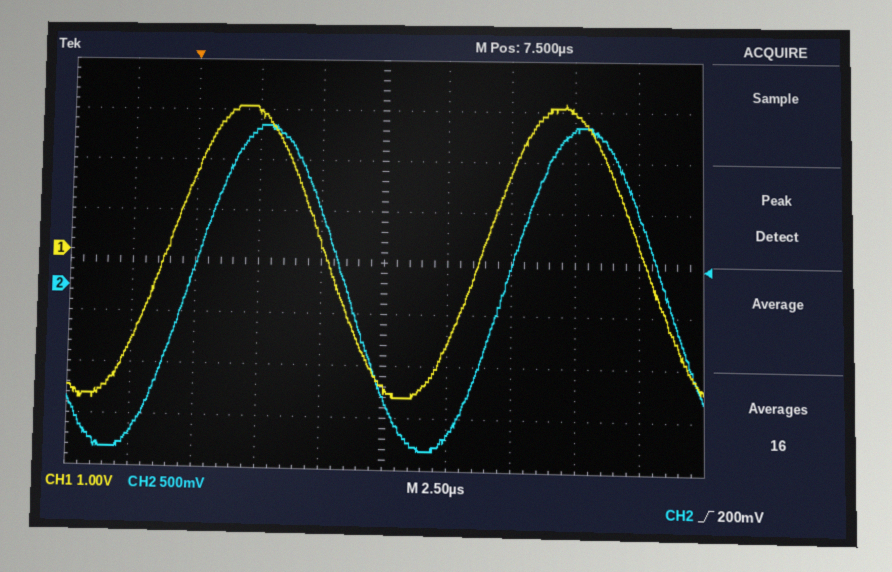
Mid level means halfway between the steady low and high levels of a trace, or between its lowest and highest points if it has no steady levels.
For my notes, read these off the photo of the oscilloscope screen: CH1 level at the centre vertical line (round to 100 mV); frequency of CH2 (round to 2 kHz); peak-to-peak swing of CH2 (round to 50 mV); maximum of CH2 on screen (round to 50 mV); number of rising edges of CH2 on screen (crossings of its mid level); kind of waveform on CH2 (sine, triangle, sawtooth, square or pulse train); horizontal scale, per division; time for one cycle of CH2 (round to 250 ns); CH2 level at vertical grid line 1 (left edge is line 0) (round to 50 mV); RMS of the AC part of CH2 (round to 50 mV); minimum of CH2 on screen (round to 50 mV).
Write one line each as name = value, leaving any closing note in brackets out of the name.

CH1 level at the centre vertical line = -2.6 V
frequency of CH2 = 80 kHz
peak-to-peak swing of CH2 = 3.15 V
maximum of CH2 on screen = 1.60 V
number of rising edges of CH2 on screen = 2
kind of waveform on CH2 = sine
horizontal scale, per division = 2.5 µs
time for one cycle of CH2 = 12.50 µs
CH2 level at vertical grid line 1 (left edge is line 0) = -1.40 V
RMS of the AC part of CH2 = 1.10 V
minimum of CH2 on screen = -1.55 V
